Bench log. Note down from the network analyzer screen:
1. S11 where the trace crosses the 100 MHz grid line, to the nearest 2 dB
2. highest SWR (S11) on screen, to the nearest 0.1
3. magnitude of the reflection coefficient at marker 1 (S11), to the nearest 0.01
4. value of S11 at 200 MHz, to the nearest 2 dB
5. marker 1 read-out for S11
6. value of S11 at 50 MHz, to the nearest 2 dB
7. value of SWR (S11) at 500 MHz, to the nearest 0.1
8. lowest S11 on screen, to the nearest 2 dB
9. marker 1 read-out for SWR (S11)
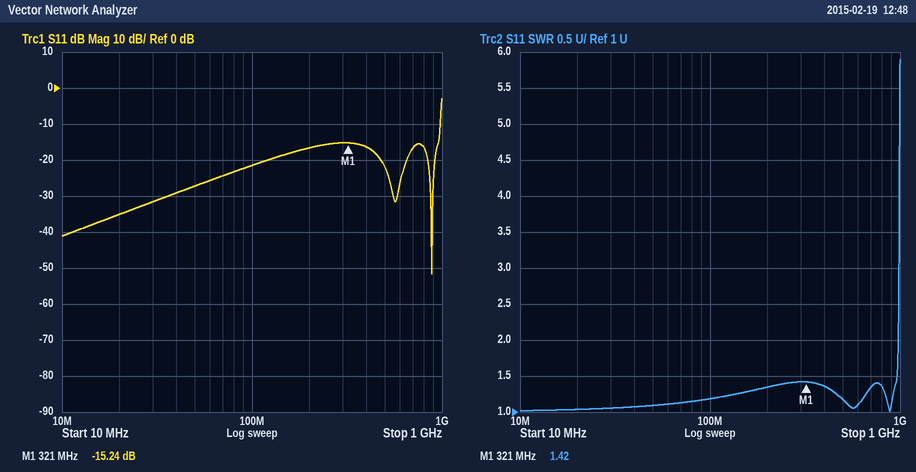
-22 dB
5.9
0.17
-16 dB
-15.24 dB
-28 dB
1.2
-52 dB
1.42
